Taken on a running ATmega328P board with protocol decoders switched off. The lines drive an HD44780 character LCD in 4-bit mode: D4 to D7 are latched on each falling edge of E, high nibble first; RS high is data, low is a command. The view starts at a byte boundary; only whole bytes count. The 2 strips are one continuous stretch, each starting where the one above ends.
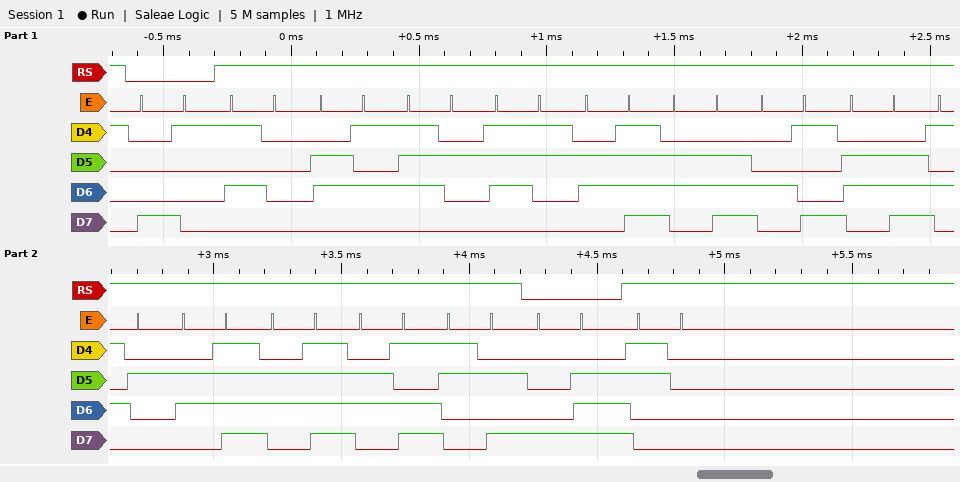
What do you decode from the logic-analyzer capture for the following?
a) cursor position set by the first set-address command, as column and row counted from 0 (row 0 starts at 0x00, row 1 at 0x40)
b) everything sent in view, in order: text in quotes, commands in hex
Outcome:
column 1, row 0
0x81 "PersonInRoom:" 0x8E "0"
